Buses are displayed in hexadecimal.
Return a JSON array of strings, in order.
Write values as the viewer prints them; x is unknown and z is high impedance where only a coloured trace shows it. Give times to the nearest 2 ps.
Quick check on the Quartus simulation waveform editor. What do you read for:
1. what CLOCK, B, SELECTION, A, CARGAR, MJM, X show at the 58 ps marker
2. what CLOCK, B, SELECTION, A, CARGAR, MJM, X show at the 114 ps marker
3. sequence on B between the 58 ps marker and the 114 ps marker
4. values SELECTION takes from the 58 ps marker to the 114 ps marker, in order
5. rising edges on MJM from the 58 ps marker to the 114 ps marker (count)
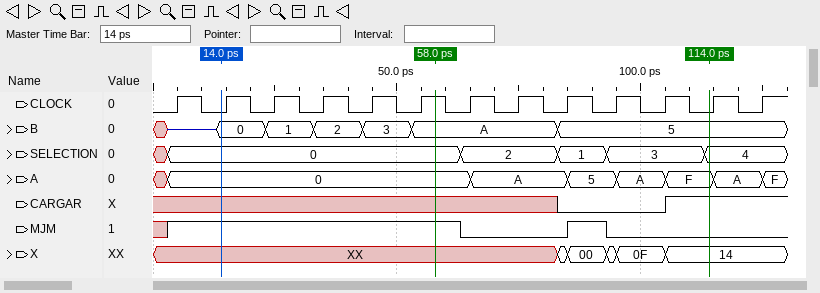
["CLOCK=1, B=A, SELECTION=0, A=0, CARGAR=x, MJM=1, X=XX", "CLOCK=0, B=5, SELECTION=4, A=F, CARGAR=1, MJM=0, X=14", "A, 5", "0, 2, 1, 3, 4", "1"]
